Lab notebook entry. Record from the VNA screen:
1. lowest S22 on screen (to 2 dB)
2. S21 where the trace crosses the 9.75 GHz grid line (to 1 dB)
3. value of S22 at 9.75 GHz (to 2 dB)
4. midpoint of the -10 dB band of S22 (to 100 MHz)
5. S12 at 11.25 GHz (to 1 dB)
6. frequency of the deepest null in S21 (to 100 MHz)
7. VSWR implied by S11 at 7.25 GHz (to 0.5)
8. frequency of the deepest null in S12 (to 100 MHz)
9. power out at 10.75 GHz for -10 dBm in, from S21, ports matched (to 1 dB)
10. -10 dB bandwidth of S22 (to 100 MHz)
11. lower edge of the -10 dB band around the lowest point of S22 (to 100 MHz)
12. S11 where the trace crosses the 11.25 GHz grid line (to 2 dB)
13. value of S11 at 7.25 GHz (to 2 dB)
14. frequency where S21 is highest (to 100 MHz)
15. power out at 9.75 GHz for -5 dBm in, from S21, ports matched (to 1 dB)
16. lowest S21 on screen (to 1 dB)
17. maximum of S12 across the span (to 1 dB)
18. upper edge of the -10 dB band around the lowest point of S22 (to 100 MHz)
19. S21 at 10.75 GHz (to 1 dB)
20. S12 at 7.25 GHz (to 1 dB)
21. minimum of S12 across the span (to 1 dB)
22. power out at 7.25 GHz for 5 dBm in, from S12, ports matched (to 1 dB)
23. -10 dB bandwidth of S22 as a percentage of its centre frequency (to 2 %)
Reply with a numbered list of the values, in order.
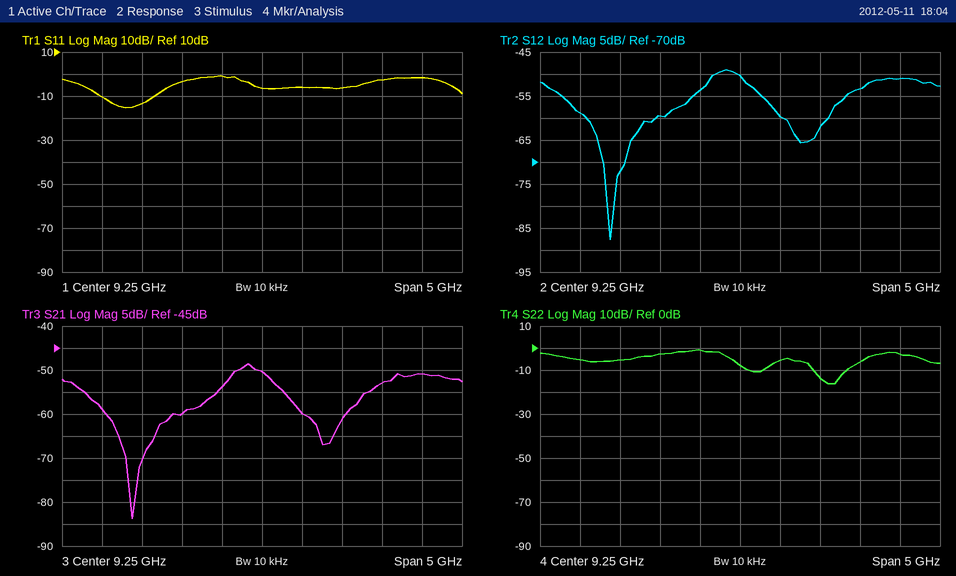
1. -16 dB
2. -60 dB
3. -6 dB
4. 10.4 GHz
5. -51 dB
6. 7.6 GHz
7. 2.0
8. 7.6 GHz
9. -63 dBm
10. 400 MHz
11. 10.2 GHz
12. -2 dB
13. -10 dB
14. 9.1 GHz
15. -65 dBm
16. -84 dB
17. -49 dB
18. 10.6 GHz
19. -53 dB
20. -59 dB
21. -88 dB
22. -54 dBm
23. 4 %
